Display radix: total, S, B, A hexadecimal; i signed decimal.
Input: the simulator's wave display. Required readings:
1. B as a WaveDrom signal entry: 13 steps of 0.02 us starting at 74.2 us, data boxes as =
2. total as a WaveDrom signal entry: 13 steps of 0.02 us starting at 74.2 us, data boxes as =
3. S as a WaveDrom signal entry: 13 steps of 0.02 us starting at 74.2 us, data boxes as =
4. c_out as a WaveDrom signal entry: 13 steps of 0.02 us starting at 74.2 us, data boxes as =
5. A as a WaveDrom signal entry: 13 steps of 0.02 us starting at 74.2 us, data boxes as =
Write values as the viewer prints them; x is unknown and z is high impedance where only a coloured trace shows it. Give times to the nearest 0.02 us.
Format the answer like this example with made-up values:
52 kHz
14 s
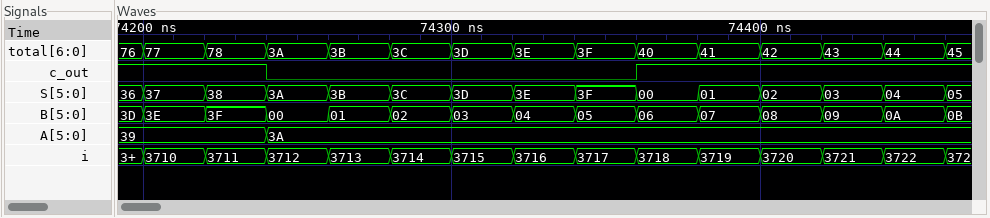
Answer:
{name: 'B', wave: '=============', data: '3E 3F 00 01 02 03 04 05 06 07 08 09 0A'}
{name: 'total', wave: '=============', data: '77 78 3A 3B 3C 3D 3E 3F 40 41 42 43 44'}
{name: 'S', wave: '=============', data: '37 38 3A 3B 3C 3D 3E 3F 00 01 02 03 04'}
{name: 'c_out', wave: '1.0.....1....'}
{name: 'A', wave: '=.=..........', data: '39 3A'}
